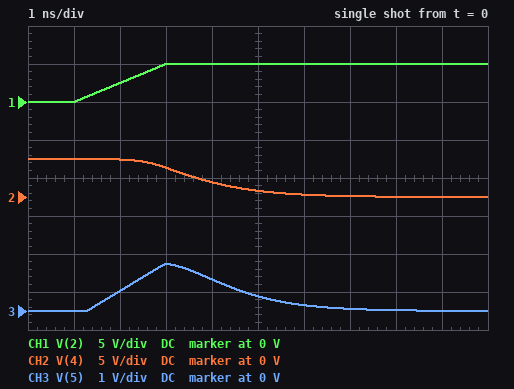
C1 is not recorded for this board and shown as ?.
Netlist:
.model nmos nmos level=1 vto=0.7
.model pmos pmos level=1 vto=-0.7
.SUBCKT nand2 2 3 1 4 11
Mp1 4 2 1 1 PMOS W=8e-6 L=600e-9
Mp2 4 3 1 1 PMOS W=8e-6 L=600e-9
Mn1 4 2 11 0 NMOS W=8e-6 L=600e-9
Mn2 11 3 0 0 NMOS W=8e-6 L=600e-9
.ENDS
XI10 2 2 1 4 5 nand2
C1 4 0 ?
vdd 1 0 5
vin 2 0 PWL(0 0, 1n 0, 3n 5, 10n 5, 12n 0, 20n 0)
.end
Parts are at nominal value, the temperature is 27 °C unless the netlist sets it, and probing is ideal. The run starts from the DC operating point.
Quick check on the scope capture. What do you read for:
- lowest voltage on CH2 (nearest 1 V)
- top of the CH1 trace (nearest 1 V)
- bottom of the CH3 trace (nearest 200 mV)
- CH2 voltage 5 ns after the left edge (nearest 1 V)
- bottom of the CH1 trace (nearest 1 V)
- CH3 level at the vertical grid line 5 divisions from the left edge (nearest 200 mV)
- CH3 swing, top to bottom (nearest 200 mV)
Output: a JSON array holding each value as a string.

["0 V", "5 V", "0 V", "1 V", "0 V", "400 mV", "1.2 V"]
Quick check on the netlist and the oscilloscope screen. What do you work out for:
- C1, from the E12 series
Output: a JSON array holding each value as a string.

["560 fF"]
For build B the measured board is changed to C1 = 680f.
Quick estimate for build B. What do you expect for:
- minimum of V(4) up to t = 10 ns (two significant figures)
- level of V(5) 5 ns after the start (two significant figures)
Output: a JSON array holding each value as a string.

["21 mV", "560 mV"]
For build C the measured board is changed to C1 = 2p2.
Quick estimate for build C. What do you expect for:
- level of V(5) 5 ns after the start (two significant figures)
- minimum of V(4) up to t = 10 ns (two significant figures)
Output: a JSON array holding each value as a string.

["1.2 V", "1.4 V"]
